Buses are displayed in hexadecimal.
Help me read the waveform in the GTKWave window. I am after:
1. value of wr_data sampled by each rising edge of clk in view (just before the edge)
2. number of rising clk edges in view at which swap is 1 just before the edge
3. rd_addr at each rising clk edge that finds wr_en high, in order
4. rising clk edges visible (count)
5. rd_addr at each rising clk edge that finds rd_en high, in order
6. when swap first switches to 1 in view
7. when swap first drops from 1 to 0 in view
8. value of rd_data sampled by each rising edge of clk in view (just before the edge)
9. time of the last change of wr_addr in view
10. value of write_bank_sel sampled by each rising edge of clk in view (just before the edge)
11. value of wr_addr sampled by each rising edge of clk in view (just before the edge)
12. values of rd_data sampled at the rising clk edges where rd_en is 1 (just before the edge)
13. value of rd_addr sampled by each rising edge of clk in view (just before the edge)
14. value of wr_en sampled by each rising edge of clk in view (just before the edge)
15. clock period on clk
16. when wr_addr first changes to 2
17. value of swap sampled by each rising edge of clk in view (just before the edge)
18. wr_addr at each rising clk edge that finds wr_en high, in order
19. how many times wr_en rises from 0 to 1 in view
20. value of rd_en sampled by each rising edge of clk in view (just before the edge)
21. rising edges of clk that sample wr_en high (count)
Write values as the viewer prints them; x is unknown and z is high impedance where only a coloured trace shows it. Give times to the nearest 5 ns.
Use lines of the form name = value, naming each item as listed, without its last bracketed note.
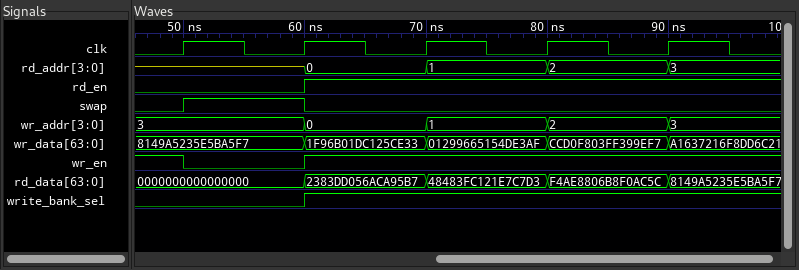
value of wr_data sampled by each rising edge of clk in view = 8149A5235E5BA5F7, 8149A5235E5BA5F7, 1F96B01DC125CE33, 01299665154DE3AF, CCD0F803FF399EF7
number of rising clk edges in view at which swap is 1 just before the edge = 1
rd_addr at each rising clk edge that finds wr_en high, in order = z, 0, 1, 2
rising clk edges visible = 5
rd_addr at each rising clk edge that finds rd_en high, in order = 0, 1, 2
when swap first switches to 1 in view = 50 ns
when swap first drops from 1 to 0 in view = 60 ns
value of rd_data sampled by each rising edge of clk in view = 0000000000000000, 0000000000000000, 2383DD056ACA95B7, 48483FC121E7C7D3, F4AE8806B8F0AC5C
time of the last change of wr_addr in view = 90 ns
value of write_bank_sel sampled by each rising edge of clk in view = 0 0 1 1 1
value of wr_addr sampled by each rising edge of clk in view = 3, 3, 0, 1, 2
values of rd_data sampled at the rising clk edges where rd_en is 1 = 2383DD056ACA95B7, 48483FC121E7C7D3, F4AE8806B8F0AC5C
value of rd_addr sampled by each rising edge of clk in view = z, z, 0, 1, 2
value of wr_en sampled by each rising edge of clk in view = 1 0 1 1 1
clock period on clk = 10 ns
when wr_addr first changes to 2 = 80 ns
value of swap sampled by each rising edge of clk in view = 0 1 0 0 0
wr_addr at each rising clk edge that finds wr_en high, in order = 3, 0, 1, 2
how many times wr_en rises from 0 to 1 in view = 1
value of rd_en sampled by each rising edge of clk in view = 0 0 1 1 1
rising edges of clk that sample wr_en high = 4
